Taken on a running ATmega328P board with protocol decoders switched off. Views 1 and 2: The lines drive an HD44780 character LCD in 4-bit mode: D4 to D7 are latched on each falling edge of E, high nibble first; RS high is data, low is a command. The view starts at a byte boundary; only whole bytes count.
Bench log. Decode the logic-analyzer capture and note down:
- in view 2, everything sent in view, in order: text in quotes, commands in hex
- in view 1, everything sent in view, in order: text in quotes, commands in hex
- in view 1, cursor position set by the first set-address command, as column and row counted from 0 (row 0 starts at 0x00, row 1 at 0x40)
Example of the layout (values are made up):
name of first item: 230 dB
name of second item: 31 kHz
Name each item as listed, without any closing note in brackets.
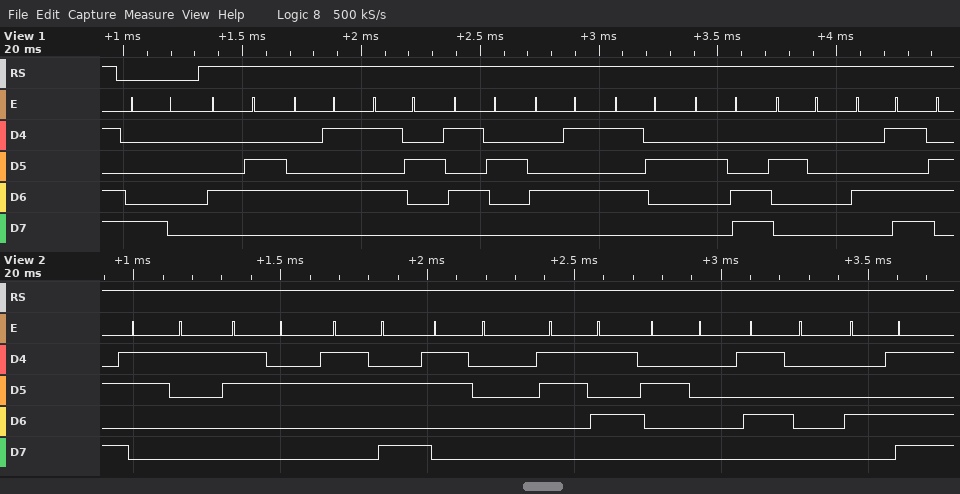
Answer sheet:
in view 2, everything sent in view, in order: text in quotes, commands in hex: "12:05 PM"
in view 1, everything sent in view, in order: text in quotes, commands in hex: 0x80 "FERRER, M"
in view 1, cursor position set by the first set-address command, as column and row counted from 0: column 0, row 0
